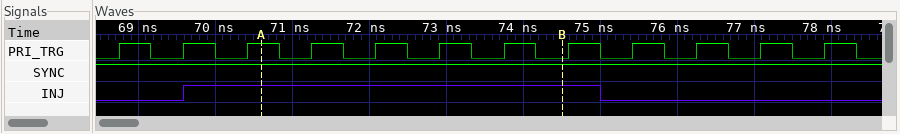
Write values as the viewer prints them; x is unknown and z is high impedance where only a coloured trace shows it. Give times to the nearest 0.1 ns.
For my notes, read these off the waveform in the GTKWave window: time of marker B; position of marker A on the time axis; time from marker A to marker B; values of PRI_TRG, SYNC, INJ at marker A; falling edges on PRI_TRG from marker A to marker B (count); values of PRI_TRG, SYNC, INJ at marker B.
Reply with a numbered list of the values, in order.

1. 74.5 ns
2. 70.6 ns
3. 3.9 ns
4. PRI_TRG=1, SYNC=1, INJ=1
5. 5
6. PRI_TRG=0, SYNC=1, INJ=1
